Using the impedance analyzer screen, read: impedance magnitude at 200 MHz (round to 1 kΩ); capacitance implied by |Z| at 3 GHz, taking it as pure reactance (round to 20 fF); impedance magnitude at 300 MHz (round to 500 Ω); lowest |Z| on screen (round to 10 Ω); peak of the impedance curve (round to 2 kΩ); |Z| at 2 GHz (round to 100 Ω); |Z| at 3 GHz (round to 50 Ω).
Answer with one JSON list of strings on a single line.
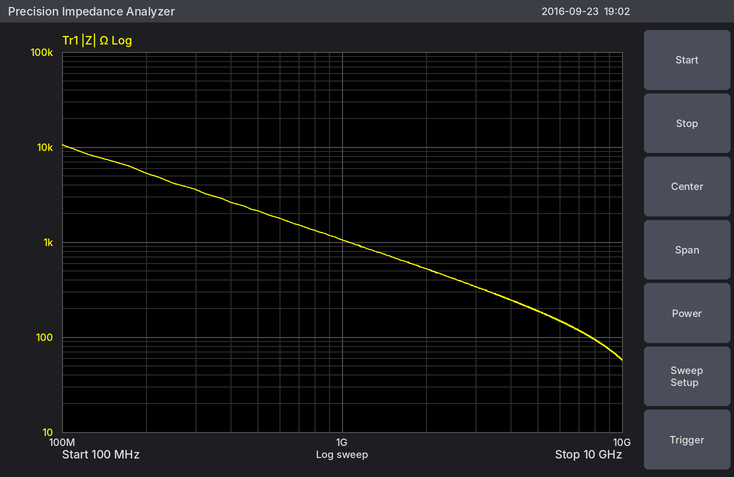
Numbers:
["5 kΩ", "160 fF", "3.5 kΩ", "60 Ω", "10 kΩ", "500 Ω", "350 Ω"]
